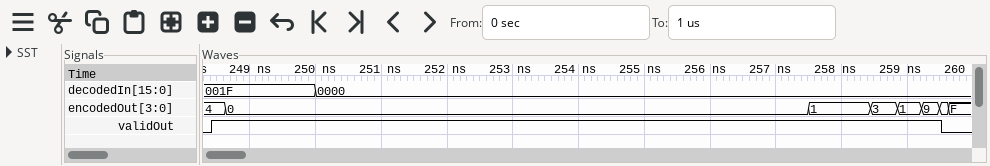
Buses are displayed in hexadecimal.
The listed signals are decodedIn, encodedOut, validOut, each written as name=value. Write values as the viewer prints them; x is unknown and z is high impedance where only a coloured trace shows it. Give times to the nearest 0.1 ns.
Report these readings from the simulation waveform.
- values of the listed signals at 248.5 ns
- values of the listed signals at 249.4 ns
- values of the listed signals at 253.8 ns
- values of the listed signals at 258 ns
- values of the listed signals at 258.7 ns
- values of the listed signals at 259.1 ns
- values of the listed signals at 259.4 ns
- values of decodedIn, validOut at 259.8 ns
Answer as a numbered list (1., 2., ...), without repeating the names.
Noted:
1. decodedIn=001F, encodedOut=4, validOut=1
2. decodedIn=001F, encodedOut=0, validOut=1
3. decodedIn=0000, encodedOut=0, validOut=1
4. decodedIn=0000, encodedOut=1, validOut=1
5. decodedIn=0000, encodedOut=3, validOut=1
6. decodedIn=0000, encodedOut=1, validOut=1
7. decodedIn=0000, encodedOut=9, validOut=1
8. decodedIn=0000, validOut=0
